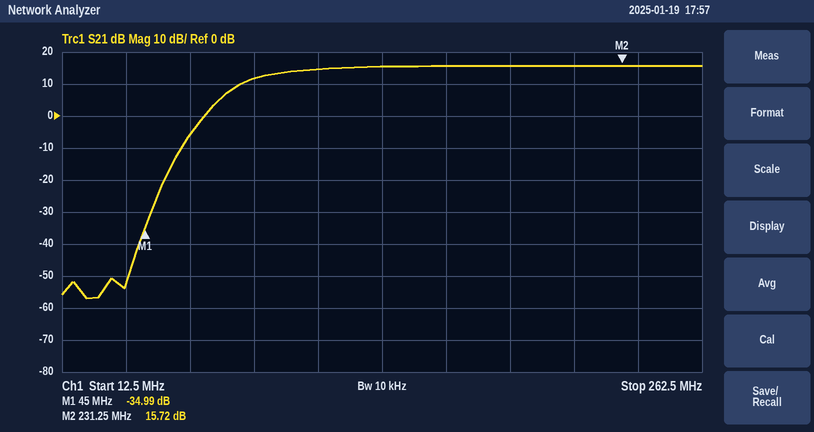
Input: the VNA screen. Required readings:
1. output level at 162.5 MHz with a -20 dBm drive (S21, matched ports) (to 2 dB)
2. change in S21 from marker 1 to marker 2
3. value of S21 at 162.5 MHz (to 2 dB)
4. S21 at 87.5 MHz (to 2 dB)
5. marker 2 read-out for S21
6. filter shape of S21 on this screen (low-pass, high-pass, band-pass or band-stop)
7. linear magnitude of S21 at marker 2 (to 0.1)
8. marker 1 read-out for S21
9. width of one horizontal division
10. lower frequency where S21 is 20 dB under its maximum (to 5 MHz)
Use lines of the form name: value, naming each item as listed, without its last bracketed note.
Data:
output level at 162.5 MHz with a -20 dBm drive (S21, matched ports): -4 dBm
change in S21 from marker 1 to marker 2: 50.71 dB
value of S21 at 162.5 MHz: 16 dB
S21 at 87.5 MHz: 12 dB
marker 2 read-out for S21: 15.72 dB
filter shape of S21 on this screen: high-pass
linear magnitude of S21 at marker 2: 6.1
marker 1 read-out for S21: -34.99 dB
width of one horizontal division: 25 MHz
lower frequency where S21 is 20 dB under its maximum: 65 MHz
